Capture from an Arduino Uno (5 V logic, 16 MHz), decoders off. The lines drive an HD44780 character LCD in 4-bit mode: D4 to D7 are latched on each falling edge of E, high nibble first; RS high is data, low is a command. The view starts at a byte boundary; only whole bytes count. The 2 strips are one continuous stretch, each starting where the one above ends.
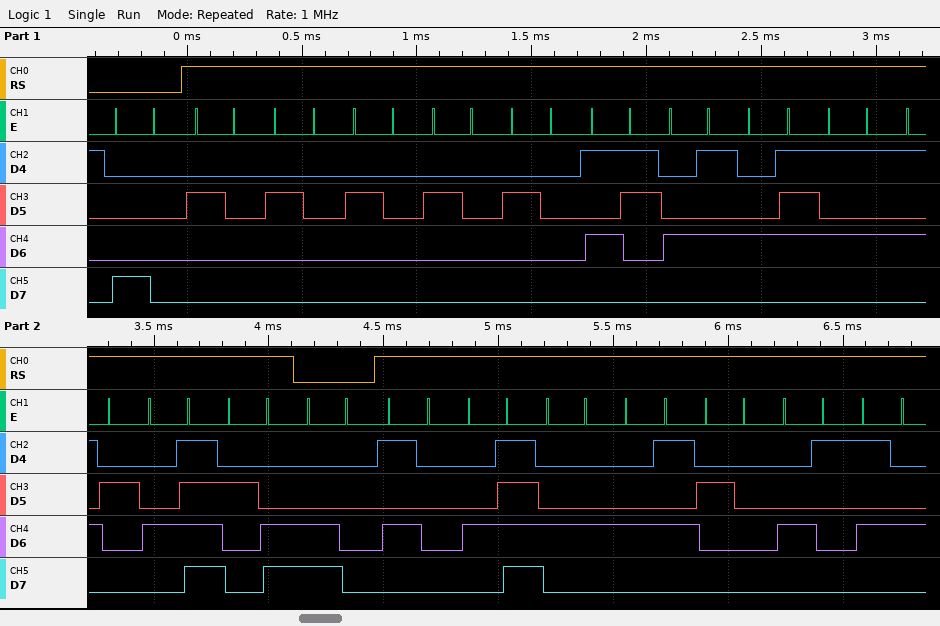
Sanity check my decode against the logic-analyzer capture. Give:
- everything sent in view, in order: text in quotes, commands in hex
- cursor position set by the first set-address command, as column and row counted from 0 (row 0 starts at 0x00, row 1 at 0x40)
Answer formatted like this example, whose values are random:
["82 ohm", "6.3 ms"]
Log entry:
["0x80 \"     SEGURO,\" 0xC0 \"PODE AT\"", "column 0, row 0"]
